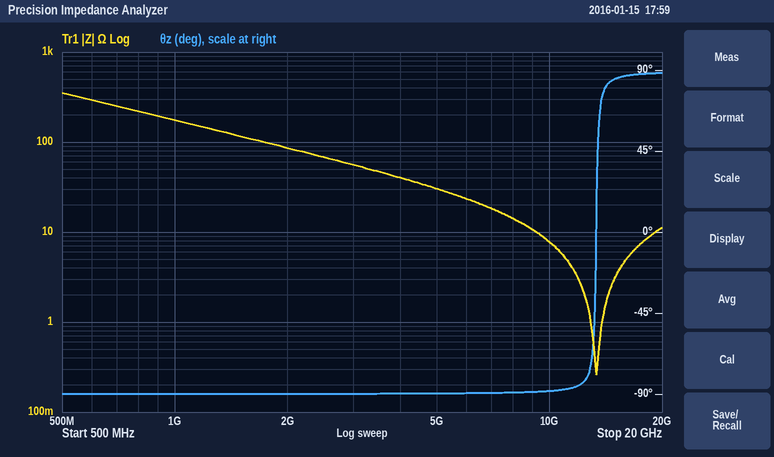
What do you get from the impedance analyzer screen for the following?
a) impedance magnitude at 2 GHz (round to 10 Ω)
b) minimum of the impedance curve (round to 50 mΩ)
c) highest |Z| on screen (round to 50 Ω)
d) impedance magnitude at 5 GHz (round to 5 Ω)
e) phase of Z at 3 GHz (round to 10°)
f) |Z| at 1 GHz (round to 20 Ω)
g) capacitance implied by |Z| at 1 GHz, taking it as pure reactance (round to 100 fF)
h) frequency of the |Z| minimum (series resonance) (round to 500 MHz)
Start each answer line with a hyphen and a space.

- 90 Ω
- 250 mΩ
- 350 Ω
- 30 Ω
- -90°
- 180 Ω
- 900 fF
- 13.5 GHz
